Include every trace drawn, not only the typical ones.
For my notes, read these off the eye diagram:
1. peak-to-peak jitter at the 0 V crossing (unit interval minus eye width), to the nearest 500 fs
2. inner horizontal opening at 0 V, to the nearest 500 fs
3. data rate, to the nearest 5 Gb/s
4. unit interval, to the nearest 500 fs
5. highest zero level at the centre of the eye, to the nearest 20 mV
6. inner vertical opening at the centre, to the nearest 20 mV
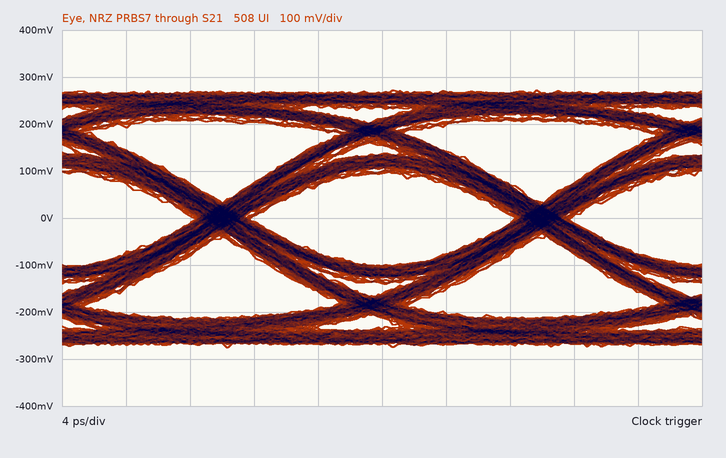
3.5 ps
16.5 ps
50 Gb/s
20.0 ps
-100 mV
200 mV
